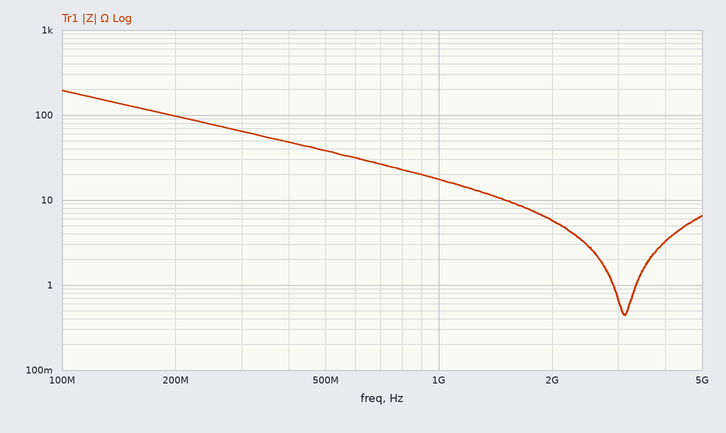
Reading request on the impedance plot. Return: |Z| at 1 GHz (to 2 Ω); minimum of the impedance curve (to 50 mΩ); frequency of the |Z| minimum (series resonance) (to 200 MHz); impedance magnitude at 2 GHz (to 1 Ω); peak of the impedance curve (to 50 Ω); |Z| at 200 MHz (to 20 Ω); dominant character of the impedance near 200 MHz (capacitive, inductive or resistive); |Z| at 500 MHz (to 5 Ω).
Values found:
18 Ω
450 mΩ
3.2 GHz
6 Ω
200 Ω
100 Ω
capacitive
40 Ω
